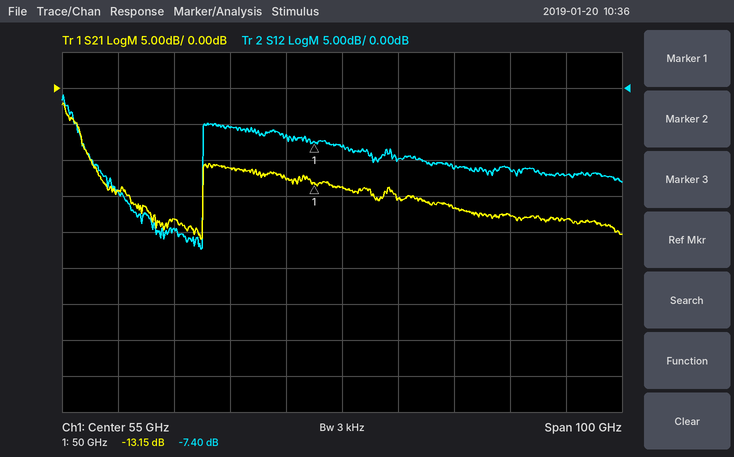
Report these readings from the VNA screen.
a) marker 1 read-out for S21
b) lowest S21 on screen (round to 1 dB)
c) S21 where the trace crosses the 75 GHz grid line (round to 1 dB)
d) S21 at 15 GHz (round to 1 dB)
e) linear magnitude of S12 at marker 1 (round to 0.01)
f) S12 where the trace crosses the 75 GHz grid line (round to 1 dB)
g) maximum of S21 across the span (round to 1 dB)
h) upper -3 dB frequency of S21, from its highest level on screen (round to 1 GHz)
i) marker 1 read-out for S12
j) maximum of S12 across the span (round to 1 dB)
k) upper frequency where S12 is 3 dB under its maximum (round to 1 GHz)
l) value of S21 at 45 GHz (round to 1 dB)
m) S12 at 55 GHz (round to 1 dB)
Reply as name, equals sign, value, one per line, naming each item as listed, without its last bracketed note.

marker 1 read-out for S21 = -13.15 dB
lowest S21 on screen = -21 dB
S21 where the trace crosses the 75 GHz grid line = -17 dB
S21 at 15 GHz = -14 dB
linear magnitude of S12 at marker 1 = 0.43
S12 where the trace crosses the 75 GHz grid line = -11 dB
maximum of S21 across the span = -2 dB
upper -3 dB frequency of S21, from its highest level on screen = 8 GHz
marker 1 read-out for S12 = -7.40 dB
maximum of S12 across the span = -1 dB
upper frequency where S12 is 3 dB under its maximum = 7 GHz
value of S21 at 45 GHz = -13 dB
S12 at 55 GHz = -8 dB
